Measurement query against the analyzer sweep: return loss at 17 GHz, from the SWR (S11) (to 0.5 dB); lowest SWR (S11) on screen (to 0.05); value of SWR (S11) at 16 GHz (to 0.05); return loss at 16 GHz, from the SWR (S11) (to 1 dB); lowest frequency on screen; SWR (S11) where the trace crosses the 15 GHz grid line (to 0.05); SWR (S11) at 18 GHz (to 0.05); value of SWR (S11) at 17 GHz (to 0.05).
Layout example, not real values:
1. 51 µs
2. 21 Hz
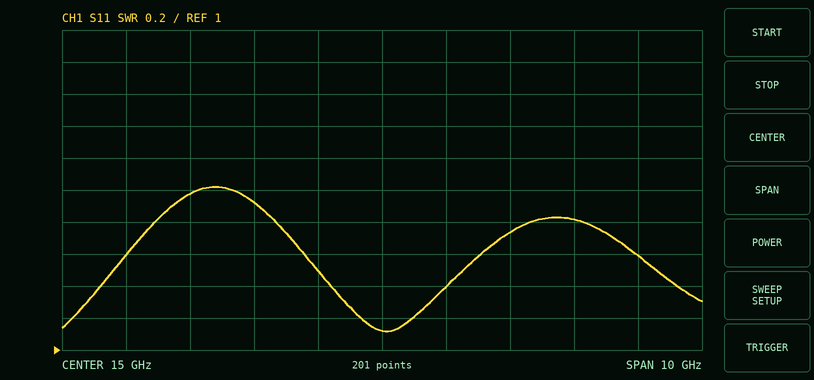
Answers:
1. 11.5 dB
2. 1.10
3. 1.40
4. 16 dB
5. 10 GHz
6. 1.10
7. 1.80
8. 1.75
